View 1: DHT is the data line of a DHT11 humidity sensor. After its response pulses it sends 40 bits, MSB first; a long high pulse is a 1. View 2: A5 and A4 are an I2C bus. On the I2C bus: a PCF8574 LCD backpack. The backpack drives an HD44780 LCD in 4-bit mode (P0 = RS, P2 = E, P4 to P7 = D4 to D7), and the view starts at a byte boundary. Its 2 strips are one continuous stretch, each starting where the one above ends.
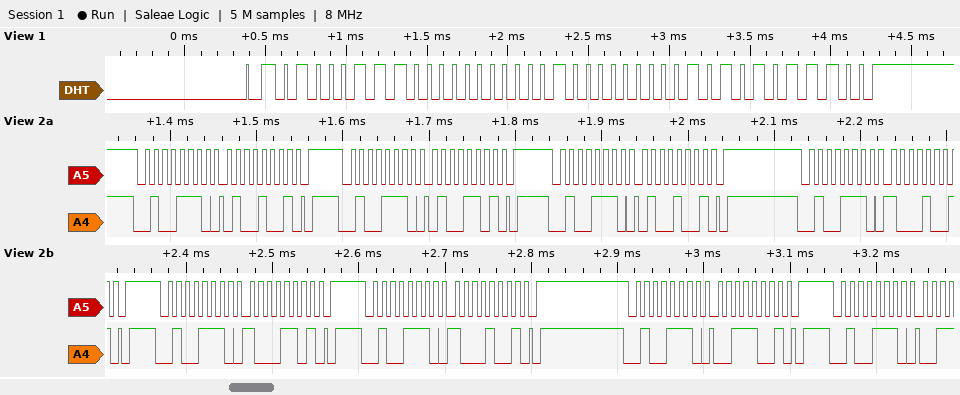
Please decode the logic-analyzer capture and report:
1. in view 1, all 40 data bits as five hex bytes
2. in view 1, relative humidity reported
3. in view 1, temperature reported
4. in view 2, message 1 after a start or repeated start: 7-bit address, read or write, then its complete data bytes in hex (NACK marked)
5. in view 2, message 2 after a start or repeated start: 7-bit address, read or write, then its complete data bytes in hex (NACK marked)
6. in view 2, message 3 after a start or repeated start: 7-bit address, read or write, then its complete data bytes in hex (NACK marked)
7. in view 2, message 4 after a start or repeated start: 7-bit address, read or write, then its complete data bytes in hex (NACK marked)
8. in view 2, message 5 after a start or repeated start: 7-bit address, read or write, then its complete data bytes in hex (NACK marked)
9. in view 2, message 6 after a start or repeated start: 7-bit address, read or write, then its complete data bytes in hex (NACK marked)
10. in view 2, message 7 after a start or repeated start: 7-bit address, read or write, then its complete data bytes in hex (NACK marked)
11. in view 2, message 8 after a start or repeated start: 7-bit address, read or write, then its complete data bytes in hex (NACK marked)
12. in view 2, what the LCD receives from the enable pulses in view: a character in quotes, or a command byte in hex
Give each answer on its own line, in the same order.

47 00 10 05 5C
71 %
16.5 °C
0x27 write: 49
0x27 write: 4D
0x27 write: 49
0x27 write: 89
0x27 write: 8D
0x27 write: 89
0x27 write: 39
0x27 write
'H'
